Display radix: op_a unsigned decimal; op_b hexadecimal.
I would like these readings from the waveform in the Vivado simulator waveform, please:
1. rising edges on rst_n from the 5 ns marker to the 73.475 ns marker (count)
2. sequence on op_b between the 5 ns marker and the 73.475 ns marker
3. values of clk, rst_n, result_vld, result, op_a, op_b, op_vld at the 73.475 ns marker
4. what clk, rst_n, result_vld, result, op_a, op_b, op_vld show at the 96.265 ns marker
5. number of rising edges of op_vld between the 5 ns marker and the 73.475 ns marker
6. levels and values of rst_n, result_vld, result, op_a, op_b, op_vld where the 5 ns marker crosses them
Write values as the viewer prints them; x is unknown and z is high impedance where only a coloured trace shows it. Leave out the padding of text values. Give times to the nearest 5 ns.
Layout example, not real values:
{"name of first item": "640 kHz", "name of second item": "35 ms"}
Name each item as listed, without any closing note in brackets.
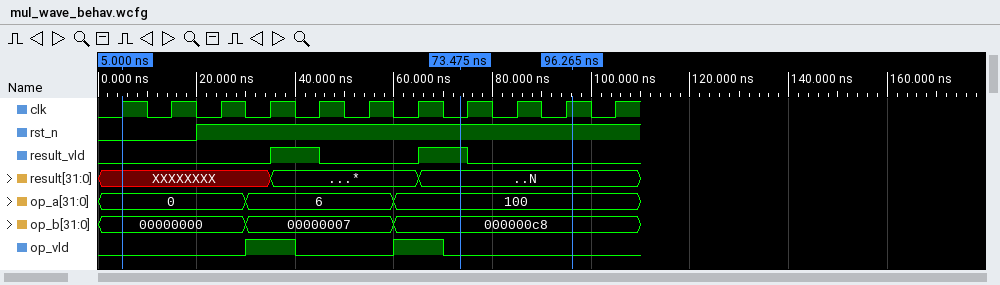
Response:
{"rising edges on rst_n from the 5 ns marker to the 73.475 ns marker": "1", "sequence on op_b between the 5 ns marker and the 73.475 ns marker": "00000000, 00000007, 000000c8", "values of clk, rst_n, result_vld, result, op_a, op_b, op_vld at the 73.475 ns marker": "clk=0, rst_n=1, result_vld=1, result=N, op_a=100, op_b=000000c8, op_vld=0", "what clk, rst_n, result_vld, result, op_a, op_b, op_vld show at the 96.265 ns marker": "clk=1, rst_n=1, result_vld=0, result=N, op_a=100, op_b=000000c8, op_vld=0", "number of rising edges of op_vld between the 5 ns marker and the 73.475 ns marker": "2", "levels and values of rst_n, result_vld, result, op_a, op_b, op_vld where the 5 ns marker crosses them": "rst_n=0, result_vld=0, result=XXXXXXXX, op_a=0, op_b=00000000, op_vld=0"}
